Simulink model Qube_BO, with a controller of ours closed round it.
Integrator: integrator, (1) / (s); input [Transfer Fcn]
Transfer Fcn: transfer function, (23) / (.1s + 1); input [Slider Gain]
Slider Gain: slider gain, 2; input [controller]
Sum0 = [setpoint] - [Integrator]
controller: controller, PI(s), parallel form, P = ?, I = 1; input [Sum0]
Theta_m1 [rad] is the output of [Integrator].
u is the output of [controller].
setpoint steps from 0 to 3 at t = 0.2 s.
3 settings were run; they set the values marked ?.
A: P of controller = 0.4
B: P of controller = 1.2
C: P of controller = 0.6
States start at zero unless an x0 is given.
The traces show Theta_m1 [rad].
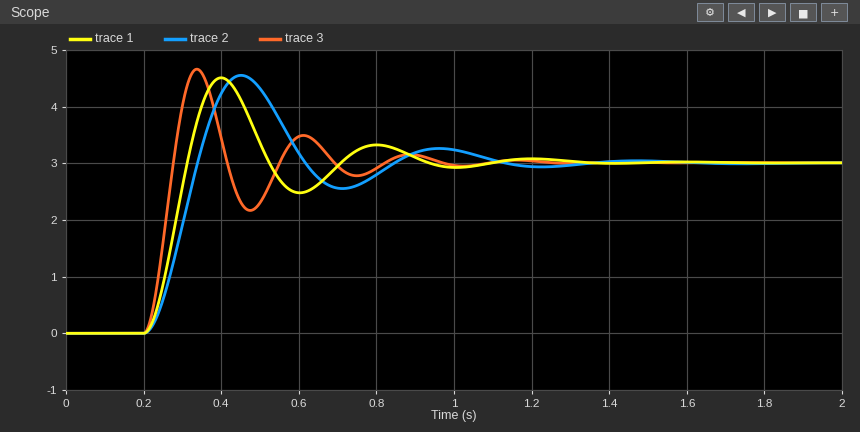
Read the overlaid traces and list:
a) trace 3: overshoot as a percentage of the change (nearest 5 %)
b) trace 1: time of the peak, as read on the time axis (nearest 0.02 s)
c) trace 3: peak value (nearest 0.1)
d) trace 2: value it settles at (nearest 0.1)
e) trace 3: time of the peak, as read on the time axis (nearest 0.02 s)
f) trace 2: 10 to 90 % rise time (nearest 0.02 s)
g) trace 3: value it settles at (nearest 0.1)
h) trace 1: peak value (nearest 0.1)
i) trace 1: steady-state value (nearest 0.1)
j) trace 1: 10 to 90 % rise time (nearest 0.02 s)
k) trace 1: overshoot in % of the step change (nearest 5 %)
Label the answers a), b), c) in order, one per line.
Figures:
a) 55 %
b) 0.40 s
c) 4.7
d) 3.0
e) 0.34 s
f) 0.10 s
g) 3.0
h) 4.5
i) 3.0
j) 0.08 s
k) 50 %
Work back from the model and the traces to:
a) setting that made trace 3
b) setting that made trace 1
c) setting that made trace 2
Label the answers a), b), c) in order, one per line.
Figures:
a) B
b) C
c) A
